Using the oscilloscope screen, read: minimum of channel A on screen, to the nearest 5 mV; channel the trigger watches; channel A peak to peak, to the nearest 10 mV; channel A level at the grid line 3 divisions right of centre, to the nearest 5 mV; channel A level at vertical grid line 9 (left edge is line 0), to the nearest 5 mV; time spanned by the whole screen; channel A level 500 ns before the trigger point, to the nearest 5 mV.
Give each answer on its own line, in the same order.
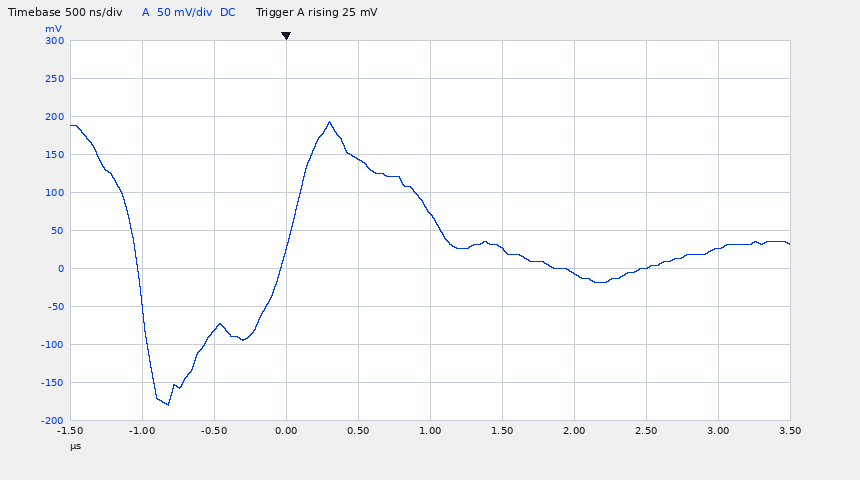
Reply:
-180 mV
channel A
370 mV
0 mV
25 mV
5 µs
-80 mV
